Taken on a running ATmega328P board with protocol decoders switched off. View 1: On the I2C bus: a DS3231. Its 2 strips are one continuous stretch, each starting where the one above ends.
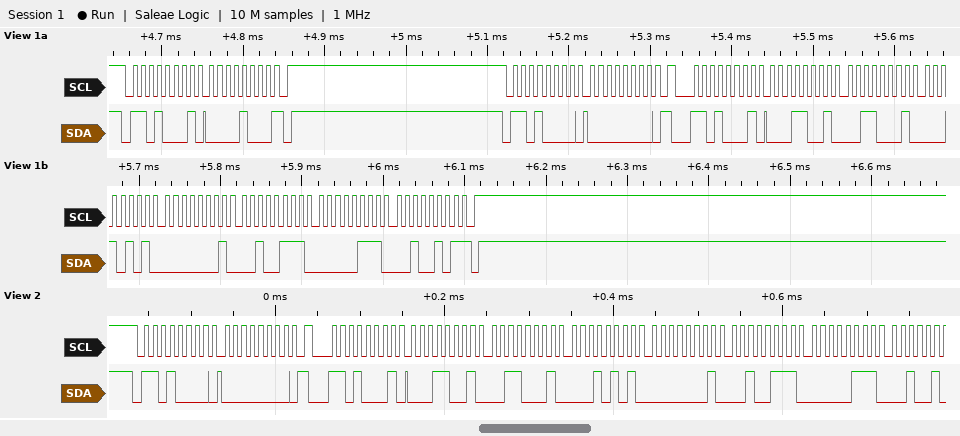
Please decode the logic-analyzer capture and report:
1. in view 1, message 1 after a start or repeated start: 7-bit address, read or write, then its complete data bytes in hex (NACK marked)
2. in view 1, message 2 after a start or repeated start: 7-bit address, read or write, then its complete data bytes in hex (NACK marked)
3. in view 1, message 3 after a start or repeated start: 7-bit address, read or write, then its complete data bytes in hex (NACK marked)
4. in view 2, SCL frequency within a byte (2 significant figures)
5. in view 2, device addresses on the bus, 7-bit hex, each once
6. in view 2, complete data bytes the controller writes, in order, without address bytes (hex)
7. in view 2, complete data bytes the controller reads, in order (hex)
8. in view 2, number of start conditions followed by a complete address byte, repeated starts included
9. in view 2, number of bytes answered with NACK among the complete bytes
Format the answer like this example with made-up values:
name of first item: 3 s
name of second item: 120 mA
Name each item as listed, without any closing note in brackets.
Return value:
in view 1, message 1 after a start or repeated start: 7-bit address, read or write, then its complete data bytes in hex: 0x68 read: 08 NACK
in view 1, message 2 after a start or repeated start: 7-bit address, read or write, then its complete data bytes in hex: 0x68 write: 00
in view 1, message 3 after a start or repeated start: 7-bit address, read or write, then its complete data bytes in hex: 0x68 read: 19 31 15 01 27 07 25 NACK
in view 2, SCL frequency within a byte: 100 kHz
in view 2, device addresses on the bus, 7-bit hex, each once: 0x68
in view 2, complete data bytes the controller writes, in order, without address bytes: 00
in view 2, complete data bytes the controller reads, in order: 19 31 15 01 27 07
in view 2, number of start conditions followed by a complete address byte, repeated starts included: 2
in view 2, number of bytes answered with NACK among the complete bytes: 0
